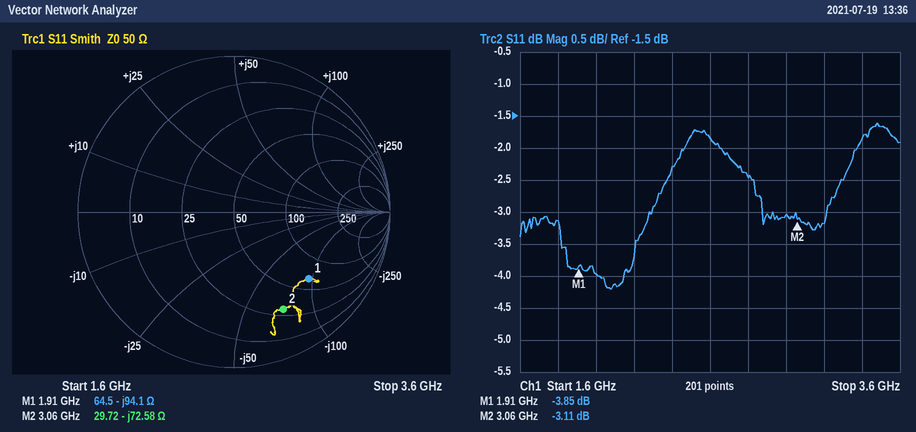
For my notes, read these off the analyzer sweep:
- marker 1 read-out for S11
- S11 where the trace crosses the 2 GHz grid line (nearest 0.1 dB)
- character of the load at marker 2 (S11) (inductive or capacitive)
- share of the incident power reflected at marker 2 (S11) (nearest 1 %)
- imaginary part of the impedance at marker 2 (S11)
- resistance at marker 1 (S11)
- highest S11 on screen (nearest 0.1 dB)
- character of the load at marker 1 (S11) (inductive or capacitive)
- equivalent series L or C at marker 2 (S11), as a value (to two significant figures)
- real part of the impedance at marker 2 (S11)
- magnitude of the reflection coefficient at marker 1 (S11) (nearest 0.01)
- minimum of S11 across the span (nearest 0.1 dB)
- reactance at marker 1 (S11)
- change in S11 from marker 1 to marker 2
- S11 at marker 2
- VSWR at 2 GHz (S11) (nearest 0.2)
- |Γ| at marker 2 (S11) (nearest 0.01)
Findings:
-3.85 dB
-4.0 dB
capacitive
49 %
-72.58 Ω
64.5 Ω
-1.6 dB
capacitive
720 fF
29.72 Ω
0.64
-4.2 dB
-94.1 Ω
0.74 dB
-3.11 dB
4.4
0.70
